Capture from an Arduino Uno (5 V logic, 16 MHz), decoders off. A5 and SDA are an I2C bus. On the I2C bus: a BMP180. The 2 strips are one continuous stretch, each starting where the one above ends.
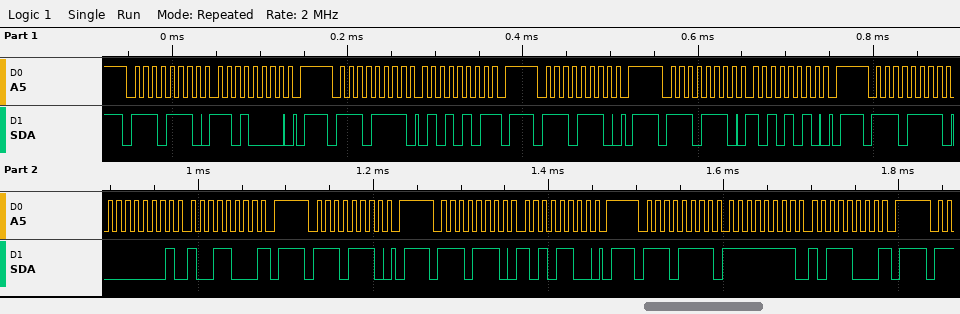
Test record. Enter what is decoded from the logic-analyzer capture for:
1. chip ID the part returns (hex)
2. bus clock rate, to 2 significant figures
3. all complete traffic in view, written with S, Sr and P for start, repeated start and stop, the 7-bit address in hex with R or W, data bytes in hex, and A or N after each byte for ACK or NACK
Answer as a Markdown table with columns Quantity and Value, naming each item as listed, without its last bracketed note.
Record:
| Quantity | Value |
|---|---|
| chip ID the part returns | 0x55 |
| bus clock rate, to 2 significant figures | 100 kHz |
| all complete traffic in view, written with S, Sr and P for start, repeated start and stop, the 7-bit address in hex with R or W, data bytes in hex, and A or N after each byte for ACK or NACK | S 77W A D0 A P S 77R A 55 N P S 77W A P S 77W A AA A P S 77R A 01 A 98 N P S 77W A P S 77W A AC A P S 77R A FF A B8 N P |
